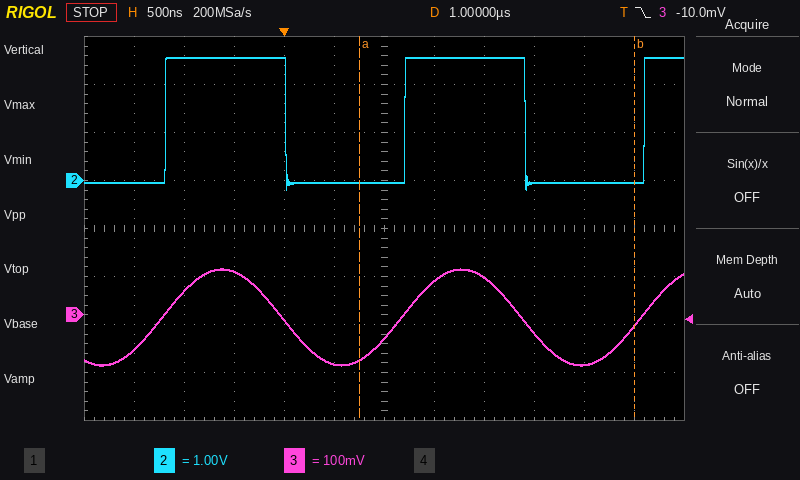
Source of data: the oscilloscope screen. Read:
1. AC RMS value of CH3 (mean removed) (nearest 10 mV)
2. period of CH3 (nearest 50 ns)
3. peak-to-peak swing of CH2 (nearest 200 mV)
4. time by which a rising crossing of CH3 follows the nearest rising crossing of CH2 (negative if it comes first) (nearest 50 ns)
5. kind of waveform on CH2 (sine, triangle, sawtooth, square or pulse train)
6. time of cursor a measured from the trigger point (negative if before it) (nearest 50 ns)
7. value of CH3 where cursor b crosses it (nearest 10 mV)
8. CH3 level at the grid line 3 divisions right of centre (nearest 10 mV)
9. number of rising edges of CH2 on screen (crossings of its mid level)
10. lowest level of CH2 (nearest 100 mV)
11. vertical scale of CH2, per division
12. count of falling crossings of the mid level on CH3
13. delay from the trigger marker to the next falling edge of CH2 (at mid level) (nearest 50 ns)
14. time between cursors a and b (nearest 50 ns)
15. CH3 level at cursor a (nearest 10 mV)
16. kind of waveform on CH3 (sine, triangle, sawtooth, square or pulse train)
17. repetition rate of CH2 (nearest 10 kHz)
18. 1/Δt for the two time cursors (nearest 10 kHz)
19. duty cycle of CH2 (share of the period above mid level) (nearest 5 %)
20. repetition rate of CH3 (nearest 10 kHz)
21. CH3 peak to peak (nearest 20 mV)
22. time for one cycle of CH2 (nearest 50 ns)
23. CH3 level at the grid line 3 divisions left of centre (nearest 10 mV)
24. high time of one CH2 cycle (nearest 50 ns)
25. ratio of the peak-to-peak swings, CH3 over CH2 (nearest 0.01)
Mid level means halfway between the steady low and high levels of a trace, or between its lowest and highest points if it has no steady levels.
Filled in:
70 mV
2.40 µs
2.8 V
-50 ns
square
+750 ns
-20 mV
-40 mV
3
-200 mV
1 V
2
2.40 µs
2.75 µs
-90 mV
sine
420 kHz
360 kHz
50 %
420 kHz
200 mV
2.40 µs
90 mV
1.20 µs
0.07
